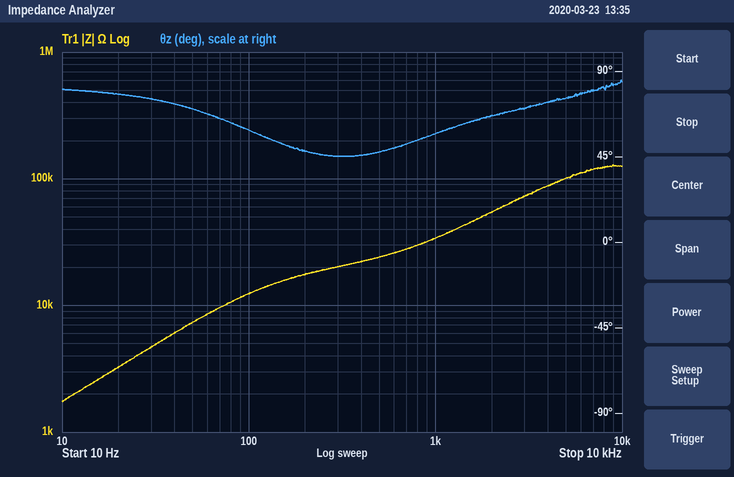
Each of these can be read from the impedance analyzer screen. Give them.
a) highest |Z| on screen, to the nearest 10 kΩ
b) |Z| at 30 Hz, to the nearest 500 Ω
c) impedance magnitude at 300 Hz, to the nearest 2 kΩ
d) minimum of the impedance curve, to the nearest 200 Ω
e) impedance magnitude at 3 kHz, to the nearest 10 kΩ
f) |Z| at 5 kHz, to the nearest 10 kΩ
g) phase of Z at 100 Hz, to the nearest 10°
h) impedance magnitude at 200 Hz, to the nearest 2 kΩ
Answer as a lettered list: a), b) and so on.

a) 130 kΩ
b) 4.5 kΩ
c) 20 kΩ
d) 1.8 kΩ
e) 70 kΩ
f) 100 kΩ
g) 60°
h) 18 kΩ
